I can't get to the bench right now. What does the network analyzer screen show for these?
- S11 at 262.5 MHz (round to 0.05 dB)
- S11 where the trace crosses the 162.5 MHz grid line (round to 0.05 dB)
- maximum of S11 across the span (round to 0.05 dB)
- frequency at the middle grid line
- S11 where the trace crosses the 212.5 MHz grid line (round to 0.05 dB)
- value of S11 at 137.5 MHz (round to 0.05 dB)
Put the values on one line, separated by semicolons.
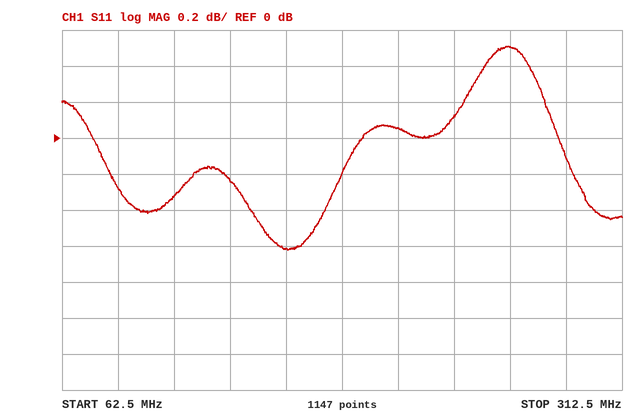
0.50 dB; -0.60 dB; 0.50 dB; 187.5 MHz; 0.05 dB; -0.25 dB
